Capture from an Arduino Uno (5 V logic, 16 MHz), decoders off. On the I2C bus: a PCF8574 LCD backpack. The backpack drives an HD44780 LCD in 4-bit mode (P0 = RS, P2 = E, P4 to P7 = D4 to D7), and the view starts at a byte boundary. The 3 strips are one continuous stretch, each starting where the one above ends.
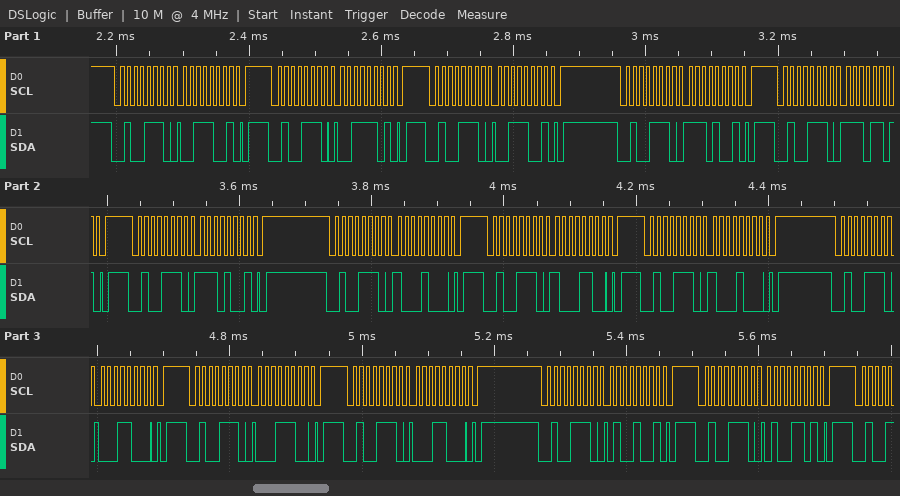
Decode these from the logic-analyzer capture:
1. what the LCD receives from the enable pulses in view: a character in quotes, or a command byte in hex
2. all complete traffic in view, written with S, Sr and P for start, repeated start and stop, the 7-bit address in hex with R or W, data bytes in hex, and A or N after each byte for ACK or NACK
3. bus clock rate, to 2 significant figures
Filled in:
'>' 0x81
S 27W A 39 A P S 27W A 3D A P S 27W A 39 A P S 27W A E9 A P S 27W A ED A P S 27W A E9 A P S 27W A 88 A P S 27W A 8C A P S 27W A 88 A P S 27W A 18 A P S 27W A 1C A P S 27W A 18 A P S 27W A 49 A P S 27W A 4D A P
100 kHz
